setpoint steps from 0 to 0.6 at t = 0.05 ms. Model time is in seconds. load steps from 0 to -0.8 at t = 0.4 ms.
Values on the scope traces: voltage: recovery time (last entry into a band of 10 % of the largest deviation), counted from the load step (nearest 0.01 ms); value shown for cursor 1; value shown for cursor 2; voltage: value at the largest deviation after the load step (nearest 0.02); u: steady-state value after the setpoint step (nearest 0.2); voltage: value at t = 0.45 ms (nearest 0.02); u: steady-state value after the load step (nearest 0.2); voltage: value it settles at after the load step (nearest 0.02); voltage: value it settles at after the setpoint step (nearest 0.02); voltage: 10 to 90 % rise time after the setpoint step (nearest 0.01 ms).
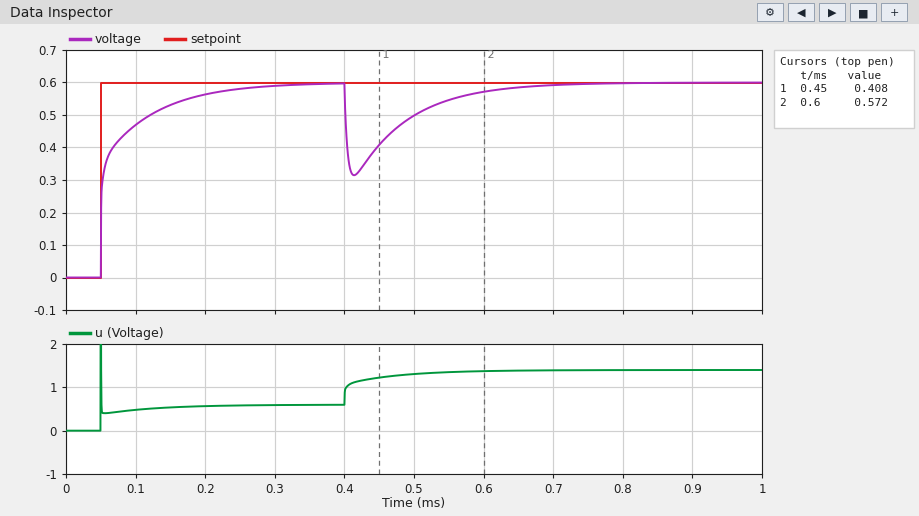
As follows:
0.20 ms
0.408
0.572
0.32
0.6
0.40
1.4
0.60
0.60
0.11 ms
